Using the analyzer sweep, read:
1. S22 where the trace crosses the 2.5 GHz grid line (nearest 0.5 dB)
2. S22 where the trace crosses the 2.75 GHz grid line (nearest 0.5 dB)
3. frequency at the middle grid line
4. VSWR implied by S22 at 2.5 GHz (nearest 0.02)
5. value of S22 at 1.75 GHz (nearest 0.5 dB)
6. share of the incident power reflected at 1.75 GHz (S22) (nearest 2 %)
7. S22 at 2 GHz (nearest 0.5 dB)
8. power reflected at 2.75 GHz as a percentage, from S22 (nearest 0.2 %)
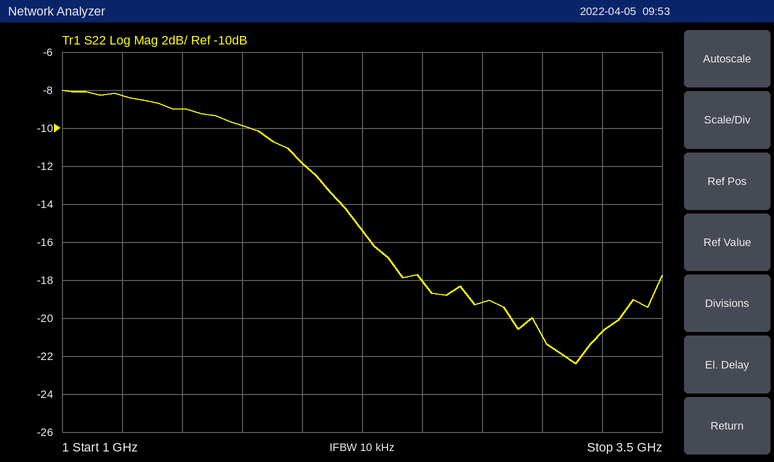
-18.0 dB
-19.0 dB
2.25 GHz
1.28
-10.0 dB
10 %
-12.0 dB
1.2 %
